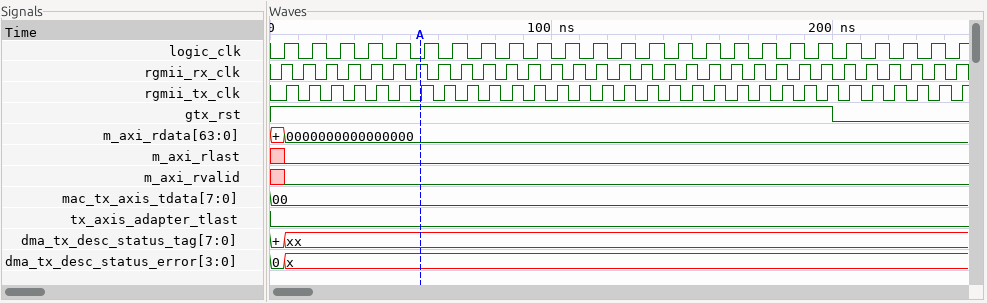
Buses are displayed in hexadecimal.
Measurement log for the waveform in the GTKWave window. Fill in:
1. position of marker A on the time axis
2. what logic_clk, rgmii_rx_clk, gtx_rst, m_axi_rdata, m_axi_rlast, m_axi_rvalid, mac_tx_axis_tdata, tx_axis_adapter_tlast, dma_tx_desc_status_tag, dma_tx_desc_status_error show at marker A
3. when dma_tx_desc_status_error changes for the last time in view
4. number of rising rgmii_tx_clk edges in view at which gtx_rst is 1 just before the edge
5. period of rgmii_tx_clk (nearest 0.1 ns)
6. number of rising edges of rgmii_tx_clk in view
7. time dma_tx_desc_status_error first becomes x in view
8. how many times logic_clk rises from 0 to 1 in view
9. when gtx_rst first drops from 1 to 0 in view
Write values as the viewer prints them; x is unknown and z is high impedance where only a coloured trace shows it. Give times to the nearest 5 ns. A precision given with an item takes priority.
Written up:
55 ns
logic_clk=0, rgmii_rx_clk=1, gtx_rst=1, m_axi_rdata=0000000000000000, m_axi_rlast=0, m_axi_rvalid=0, mac_tx_axis_tdata=00, tx_axis_adapter_tlast=0, dma_tx_desc_status_tag=xx, dma_tx_desc_status_error=x
5 ns
25
8 ns
31
5 ns
25
200 ns
